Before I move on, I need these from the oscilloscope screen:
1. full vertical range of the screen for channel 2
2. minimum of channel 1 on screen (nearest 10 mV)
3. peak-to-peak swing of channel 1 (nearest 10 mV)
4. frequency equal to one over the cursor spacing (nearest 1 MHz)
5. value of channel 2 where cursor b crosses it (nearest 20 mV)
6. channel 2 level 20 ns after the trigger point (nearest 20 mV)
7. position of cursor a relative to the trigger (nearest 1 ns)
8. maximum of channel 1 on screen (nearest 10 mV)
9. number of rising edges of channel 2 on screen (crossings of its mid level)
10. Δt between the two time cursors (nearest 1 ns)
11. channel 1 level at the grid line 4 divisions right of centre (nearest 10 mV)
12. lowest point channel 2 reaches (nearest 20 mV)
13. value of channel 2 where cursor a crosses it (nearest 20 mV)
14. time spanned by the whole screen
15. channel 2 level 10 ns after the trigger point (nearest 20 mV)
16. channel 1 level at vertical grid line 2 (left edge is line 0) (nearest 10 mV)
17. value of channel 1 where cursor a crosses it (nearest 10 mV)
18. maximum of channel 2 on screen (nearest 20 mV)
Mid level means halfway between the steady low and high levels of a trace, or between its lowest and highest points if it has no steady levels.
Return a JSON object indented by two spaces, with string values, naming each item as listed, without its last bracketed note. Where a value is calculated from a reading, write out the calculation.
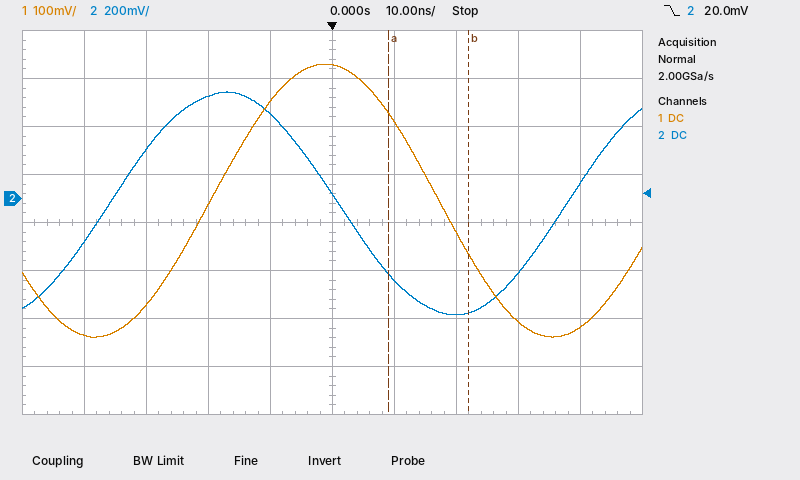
{
  "full vertical range of the screen for channel 2": "1.6 V",
  "minimum of channel 1 on screen": "-290 mV",
  "peak-to-peak swing of channel 1": "280 mV − (-290 mV) = 570 mV",
  "frequency equal to one over the cursor spacing": "1 / 13 ns ≈ 77 MHz",
  "value of channel 2 where cursor b crosses it": "-480 mV",
  "channel 2 level 20 ns after the trigger point": "-480 mV",
  "position of cursor a relative to the trigger": "+9 ns",
  "maximum of channel 1 on screen": "280 mV",
  "number of rising edges of channel 2 on screen": "2",
  "Δt between the two time cursors": "13 ns",
  "channel 1 level at the grid line 4 divisions right of centre": "-270 mV",
  "lowest point channel 2 reaches": "-480 mV",
  "value of channel 2 where cursor a crosses it": "-320 mV",
  "time spanned by the whole screen": "100 ns",
  "channel 2 level 10 ns after the trigger point": "-340 mV",
  "channel 1 level at vertical grid line 2 (left edge is line 0)": "-220 mV",
  "value of channel 1 where cursor a crosses it": "180 mV",
  "maximum of channel 2 on screen": "440 mV"
}
